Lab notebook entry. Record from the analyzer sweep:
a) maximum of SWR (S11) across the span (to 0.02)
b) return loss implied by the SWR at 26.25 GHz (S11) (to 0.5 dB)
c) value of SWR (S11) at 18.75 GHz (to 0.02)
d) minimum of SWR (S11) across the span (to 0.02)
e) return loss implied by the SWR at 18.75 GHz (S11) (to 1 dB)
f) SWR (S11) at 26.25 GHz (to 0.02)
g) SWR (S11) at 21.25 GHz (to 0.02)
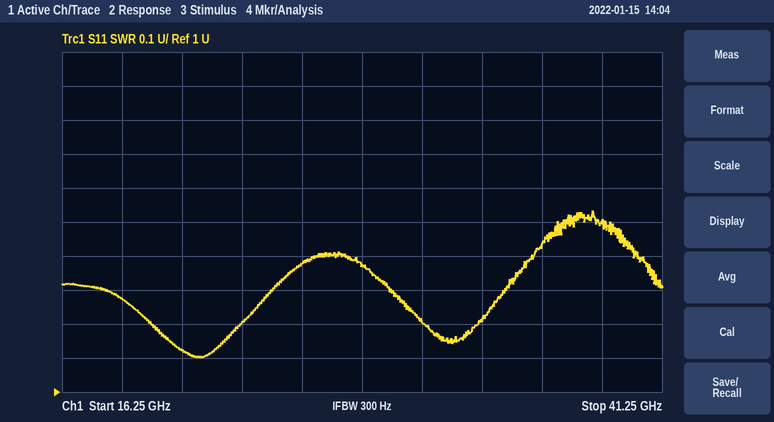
1.54
16.0 dB
1.28
1.10
18 dB
1.38
1.12
